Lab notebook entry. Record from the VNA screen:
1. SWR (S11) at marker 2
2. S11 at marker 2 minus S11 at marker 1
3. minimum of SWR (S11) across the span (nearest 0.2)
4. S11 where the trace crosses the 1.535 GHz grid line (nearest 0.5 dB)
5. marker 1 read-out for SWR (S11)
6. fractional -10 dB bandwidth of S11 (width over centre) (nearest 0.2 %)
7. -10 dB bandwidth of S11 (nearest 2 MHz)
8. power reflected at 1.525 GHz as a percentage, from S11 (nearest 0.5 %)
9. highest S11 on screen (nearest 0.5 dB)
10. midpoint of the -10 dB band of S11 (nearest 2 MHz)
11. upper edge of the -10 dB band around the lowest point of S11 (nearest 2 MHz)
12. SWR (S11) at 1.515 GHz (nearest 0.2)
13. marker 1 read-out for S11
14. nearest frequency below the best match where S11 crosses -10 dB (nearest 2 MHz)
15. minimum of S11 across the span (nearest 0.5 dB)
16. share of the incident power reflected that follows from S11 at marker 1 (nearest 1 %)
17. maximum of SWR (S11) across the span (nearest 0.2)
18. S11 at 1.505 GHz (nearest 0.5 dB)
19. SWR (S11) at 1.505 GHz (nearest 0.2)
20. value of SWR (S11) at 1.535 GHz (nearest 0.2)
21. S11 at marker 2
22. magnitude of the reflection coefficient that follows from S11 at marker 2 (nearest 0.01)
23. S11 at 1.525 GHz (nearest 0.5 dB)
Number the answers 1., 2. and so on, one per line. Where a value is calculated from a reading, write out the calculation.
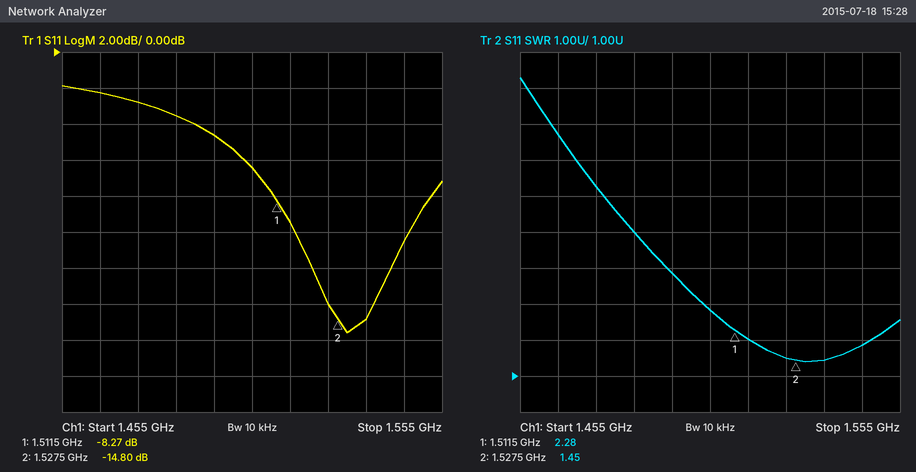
1. 1.45
2. -14.8 − (-8.27) = -6.53 dB
3. 1.4
4. -15.0 dB
5. 2.28
6. 30 MHz / 1.531 GHz ≈ 2.0 %
7. 1.546 GHz − 1.516 GHz = 30 MHz
8. 10^(-14/10) ≈ 4.0 %
9. -2.0 dB
10. 1.532 GHz
11. 1.546 GHz
12. 2.0
13. -8.27 dB
14. 1.516 GHz
15. -15.5 dB
16. 10^(-8.27/10) ≈ 15 %
17. 9.2
18. -6.5 dB
19. 2.8
20. 1.4
21. -14.80 dB
22. 10^(-14.8/20) ≈ 0.18
23. -14.0 dB
